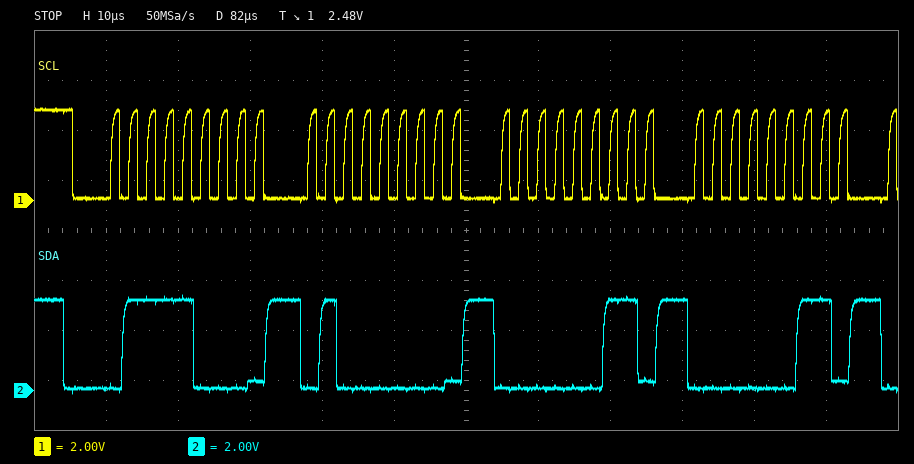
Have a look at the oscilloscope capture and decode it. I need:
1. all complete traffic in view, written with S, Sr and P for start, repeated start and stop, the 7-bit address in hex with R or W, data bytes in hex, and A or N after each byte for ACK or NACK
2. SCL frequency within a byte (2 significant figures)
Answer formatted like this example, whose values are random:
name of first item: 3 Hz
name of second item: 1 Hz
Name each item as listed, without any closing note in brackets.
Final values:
all complete traffic in view, written with S, Sr and P for start, repeated start and stop, the 7-bit address in hex with R or W, data bytes in hex, and A or N after each byte for ACK or NACK: S 3CW A 40 A 03 A 03 A
SCL frequency within a byte: 400 kHz
